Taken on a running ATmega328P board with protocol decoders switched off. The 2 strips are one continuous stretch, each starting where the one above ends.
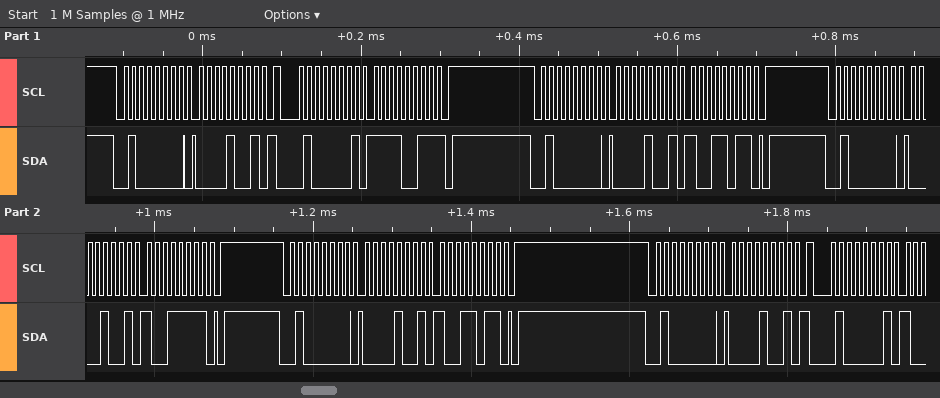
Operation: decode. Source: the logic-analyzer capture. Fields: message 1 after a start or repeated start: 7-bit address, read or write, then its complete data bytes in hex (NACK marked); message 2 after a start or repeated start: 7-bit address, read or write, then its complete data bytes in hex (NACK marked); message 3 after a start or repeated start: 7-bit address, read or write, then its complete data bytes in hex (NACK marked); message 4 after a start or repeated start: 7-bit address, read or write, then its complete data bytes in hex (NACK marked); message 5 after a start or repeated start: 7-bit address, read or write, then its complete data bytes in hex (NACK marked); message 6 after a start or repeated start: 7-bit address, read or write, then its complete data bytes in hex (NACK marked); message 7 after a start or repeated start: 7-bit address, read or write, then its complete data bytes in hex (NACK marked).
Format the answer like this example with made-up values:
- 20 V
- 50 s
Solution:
- 0x20 write: 09
- 0x20 read: F3 NACK
- 0x20 write: 09 9B
- 0x20 write: 09 9F
- 0x20 write: 09 9B
- 0x20 write: 09
- 0x20 read
